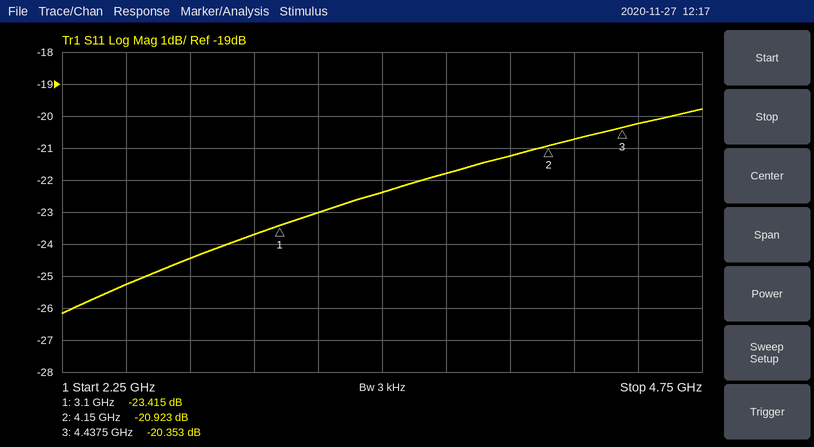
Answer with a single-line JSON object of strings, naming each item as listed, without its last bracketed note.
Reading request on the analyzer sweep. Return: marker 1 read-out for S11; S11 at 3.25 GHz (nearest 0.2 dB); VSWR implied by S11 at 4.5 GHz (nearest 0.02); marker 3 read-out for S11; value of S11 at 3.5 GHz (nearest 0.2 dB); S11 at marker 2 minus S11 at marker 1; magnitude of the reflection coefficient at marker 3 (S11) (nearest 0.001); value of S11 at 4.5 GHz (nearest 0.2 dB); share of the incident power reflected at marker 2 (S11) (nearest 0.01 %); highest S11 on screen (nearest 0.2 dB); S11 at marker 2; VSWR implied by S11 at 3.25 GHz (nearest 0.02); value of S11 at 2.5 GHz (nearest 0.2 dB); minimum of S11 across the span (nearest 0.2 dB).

{"marker 1 read-out for S11": "-23.415 dB", "S11 at 3.25 GHz": "-23.0 dB", "VSWR implied by S11 at 4.5 GHz": "1.22", "marker 3 read-out for S11": "-20.353 dB", "value of S11 at 3.5 GHz": "-22.4 dB", "S11 at marker 2 minus S11 at marker 1": "2.492 dB", "magnitude of the reflection coefficient at marker 3 (S11)": "0.096", "value of S11 at 4.5 GHz": "-20.2 dB", "share of the incident power reflected at marker 2 (S11)": "0.81 %", "highest S11 on screen": "-19.8 dB", "S11 at marker 2": "-20.923 dB", "VSWR implied by S11 at 3.25 GHz": "1.16", "value of S11 at 2.5 GHz": "-25.2 dB", "minimum of S11 across the span": "-26.2 dB"}
